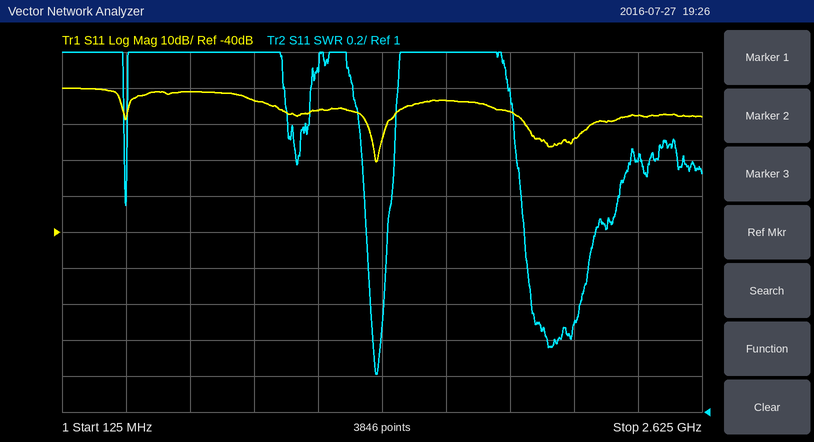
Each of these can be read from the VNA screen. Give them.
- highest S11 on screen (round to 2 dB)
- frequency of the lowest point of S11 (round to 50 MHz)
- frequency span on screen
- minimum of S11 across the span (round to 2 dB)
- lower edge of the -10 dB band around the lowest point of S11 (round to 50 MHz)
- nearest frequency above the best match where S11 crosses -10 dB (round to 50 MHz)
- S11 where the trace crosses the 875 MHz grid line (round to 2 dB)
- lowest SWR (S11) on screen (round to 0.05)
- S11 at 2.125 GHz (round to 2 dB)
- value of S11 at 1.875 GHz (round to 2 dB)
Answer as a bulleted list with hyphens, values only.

- 0 dB
- 1.35 GHz
- 2.5 GHz
- -20 dB
- 1.30 GHz
- 1.40 GHz
- -4 dB
- 1.20
- -14 dB
- -6 dB
